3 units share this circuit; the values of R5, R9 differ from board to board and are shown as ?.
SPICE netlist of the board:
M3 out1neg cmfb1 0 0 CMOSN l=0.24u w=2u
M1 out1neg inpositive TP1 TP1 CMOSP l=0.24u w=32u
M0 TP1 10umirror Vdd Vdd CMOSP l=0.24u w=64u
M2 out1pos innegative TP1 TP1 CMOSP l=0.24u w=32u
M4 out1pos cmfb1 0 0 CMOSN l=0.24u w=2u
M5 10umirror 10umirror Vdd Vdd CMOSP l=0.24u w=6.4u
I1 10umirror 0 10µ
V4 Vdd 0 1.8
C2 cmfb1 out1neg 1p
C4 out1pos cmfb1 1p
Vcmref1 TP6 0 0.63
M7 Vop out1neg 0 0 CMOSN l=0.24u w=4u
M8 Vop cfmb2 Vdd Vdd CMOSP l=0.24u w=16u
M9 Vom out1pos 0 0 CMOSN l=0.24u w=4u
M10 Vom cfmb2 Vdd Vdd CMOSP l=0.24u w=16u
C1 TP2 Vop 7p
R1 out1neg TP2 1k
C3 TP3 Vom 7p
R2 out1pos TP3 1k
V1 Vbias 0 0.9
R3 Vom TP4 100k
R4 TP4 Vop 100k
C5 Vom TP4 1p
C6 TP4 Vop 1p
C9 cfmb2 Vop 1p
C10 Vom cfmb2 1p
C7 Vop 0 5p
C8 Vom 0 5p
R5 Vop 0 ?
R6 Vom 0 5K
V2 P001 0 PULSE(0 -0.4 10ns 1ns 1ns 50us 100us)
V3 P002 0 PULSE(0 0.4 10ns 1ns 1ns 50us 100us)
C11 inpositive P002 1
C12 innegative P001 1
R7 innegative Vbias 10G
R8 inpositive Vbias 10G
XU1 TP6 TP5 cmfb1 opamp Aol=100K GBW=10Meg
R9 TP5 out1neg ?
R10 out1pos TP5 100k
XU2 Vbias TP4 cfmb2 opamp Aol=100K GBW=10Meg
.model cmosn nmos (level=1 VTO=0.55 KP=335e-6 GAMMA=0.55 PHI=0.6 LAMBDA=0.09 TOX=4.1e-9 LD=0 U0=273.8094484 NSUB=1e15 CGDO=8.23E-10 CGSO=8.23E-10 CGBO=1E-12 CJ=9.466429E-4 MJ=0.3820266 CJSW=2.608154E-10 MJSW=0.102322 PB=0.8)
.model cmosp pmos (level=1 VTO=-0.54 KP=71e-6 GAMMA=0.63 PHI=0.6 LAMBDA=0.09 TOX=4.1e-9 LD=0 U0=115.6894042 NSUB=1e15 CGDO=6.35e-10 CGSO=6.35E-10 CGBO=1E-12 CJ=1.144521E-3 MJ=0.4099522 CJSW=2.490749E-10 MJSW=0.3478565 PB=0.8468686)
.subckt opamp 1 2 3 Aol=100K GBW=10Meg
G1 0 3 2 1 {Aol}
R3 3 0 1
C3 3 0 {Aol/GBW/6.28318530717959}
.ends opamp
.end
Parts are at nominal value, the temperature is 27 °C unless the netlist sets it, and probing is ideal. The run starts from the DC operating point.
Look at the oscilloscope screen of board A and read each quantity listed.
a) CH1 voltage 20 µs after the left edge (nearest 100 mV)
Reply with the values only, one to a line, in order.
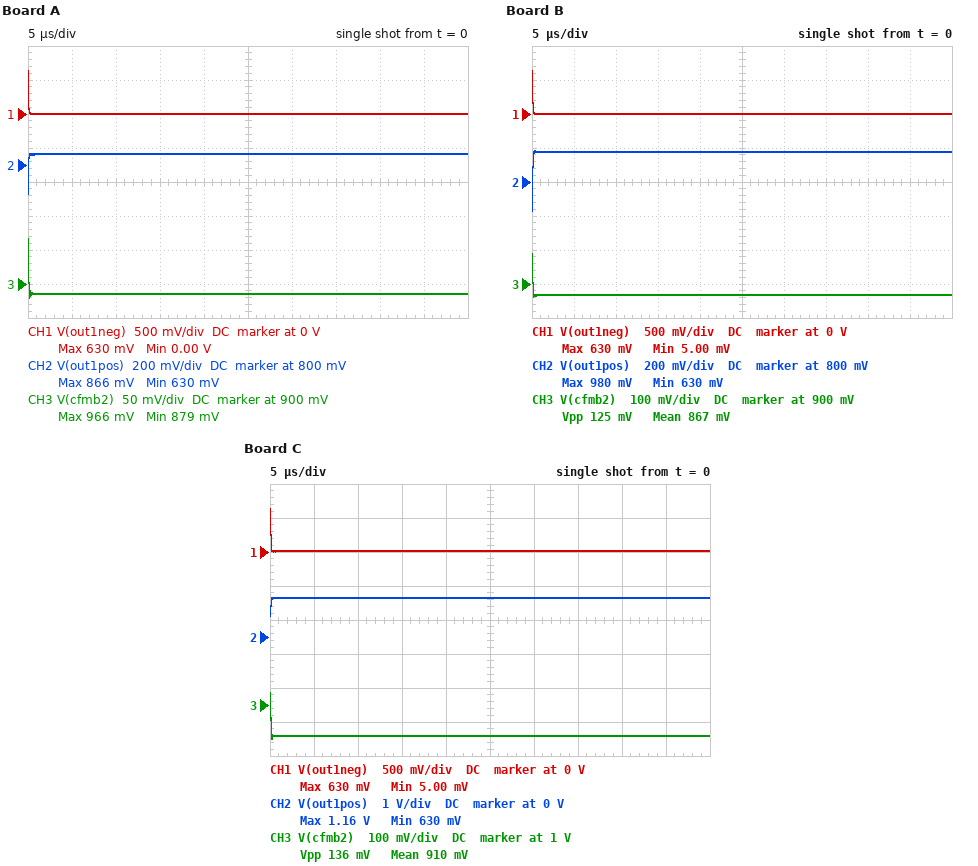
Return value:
0 V
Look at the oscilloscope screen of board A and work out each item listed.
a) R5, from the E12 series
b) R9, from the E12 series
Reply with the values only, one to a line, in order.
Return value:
3.9 kΩ
270 kΩ
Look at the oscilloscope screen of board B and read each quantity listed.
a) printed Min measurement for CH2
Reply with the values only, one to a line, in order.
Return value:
630 mV
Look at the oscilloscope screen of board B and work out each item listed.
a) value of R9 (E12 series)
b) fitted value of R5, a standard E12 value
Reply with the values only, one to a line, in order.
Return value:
180 kΩ
5.6 kΩ
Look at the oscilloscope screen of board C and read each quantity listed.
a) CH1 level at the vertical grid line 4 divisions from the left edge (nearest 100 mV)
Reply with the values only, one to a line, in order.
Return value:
0 V
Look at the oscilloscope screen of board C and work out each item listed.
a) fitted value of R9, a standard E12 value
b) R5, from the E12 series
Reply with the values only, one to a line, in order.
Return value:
120 kΩ
12 kΩ
